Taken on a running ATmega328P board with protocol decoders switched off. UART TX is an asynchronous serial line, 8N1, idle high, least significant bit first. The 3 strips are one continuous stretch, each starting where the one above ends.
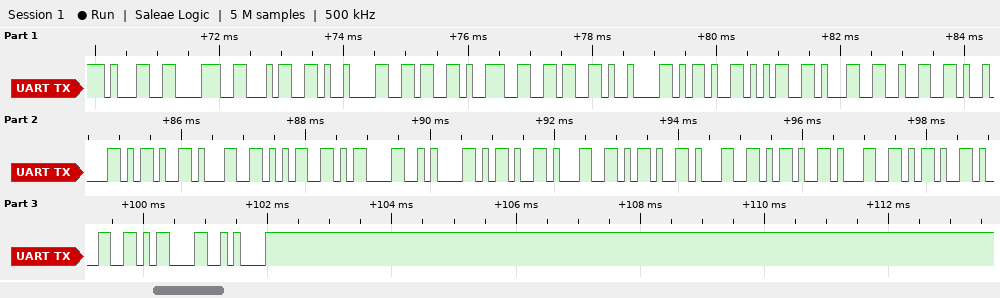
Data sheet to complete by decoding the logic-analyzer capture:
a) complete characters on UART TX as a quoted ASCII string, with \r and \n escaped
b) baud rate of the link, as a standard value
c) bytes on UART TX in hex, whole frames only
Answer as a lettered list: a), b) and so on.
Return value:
a) "184\t696\t-512\t-15\r\n-1-1-1-1\r\n"
b) 9600 baud
c) 31 38 34 09 36 39 36 09 2D 35 31 32 09 2D 31 35 0D 0A 2D 31 2D 31 2D 31 2D 31 0D 0A
